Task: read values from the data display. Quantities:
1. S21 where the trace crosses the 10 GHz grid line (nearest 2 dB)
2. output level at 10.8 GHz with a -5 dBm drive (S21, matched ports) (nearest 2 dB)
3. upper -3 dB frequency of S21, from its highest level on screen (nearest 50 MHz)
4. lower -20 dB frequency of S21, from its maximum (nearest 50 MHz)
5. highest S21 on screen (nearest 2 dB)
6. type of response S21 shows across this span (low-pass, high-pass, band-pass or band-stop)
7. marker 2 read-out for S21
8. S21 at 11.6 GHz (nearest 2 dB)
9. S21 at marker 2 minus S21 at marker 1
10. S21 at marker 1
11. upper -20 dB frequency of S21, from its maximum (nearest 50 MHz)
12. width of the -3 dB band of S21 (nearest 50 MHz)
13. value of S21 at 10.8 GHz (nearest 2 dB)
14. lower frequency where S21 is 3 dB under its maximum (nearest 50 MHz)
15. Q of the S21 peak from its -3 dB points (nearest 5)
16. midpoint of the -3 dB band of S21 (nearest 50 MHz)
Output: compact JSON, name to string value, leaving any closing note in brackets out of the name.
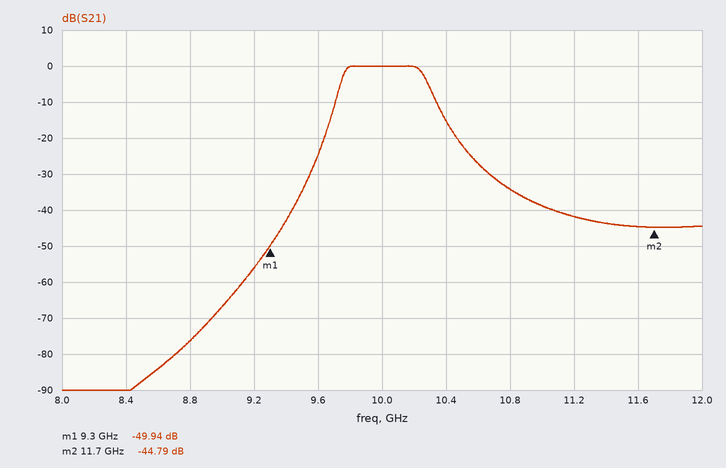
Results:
{"S21 where the trace crosses the 10 GHz grid line": "0 dB", "output level at 10.8 GHz with a -5 dBm drive (S21, matched ports)": "-40 dBm", "upper -3 dB frequency of S21, from its highest level on screen": "10.25 GHz", "lower -20 dB frequency of S21, from its maximum": "9.65 GHz", "highest S21 on screen": "0 dB", "type of response S21 shows across this span": "band-pass", "marker 2 read-out for S21": "-44.79 dB", "S21 at 11.6 GHz": "-44 dB", "S21 at marker 2 minus S21 at marker 1": "5.15 dB", "S21 at marker 1": "-49.94 dB", "upper -20 dB frequency of S21, from its maximum": "10.45 GHz", "width of the -3 dB band of S21": "500 MHz", "value of S21 at 10.8 GHz": "-34 dB", "lower frequency where S21 is 3 dB under its maximum": "9.75 GHz", "Q of the S21 peak from its -3 dB points": "20", "midpoint of the -3 dB band of S21": "10.00 GHz"}
